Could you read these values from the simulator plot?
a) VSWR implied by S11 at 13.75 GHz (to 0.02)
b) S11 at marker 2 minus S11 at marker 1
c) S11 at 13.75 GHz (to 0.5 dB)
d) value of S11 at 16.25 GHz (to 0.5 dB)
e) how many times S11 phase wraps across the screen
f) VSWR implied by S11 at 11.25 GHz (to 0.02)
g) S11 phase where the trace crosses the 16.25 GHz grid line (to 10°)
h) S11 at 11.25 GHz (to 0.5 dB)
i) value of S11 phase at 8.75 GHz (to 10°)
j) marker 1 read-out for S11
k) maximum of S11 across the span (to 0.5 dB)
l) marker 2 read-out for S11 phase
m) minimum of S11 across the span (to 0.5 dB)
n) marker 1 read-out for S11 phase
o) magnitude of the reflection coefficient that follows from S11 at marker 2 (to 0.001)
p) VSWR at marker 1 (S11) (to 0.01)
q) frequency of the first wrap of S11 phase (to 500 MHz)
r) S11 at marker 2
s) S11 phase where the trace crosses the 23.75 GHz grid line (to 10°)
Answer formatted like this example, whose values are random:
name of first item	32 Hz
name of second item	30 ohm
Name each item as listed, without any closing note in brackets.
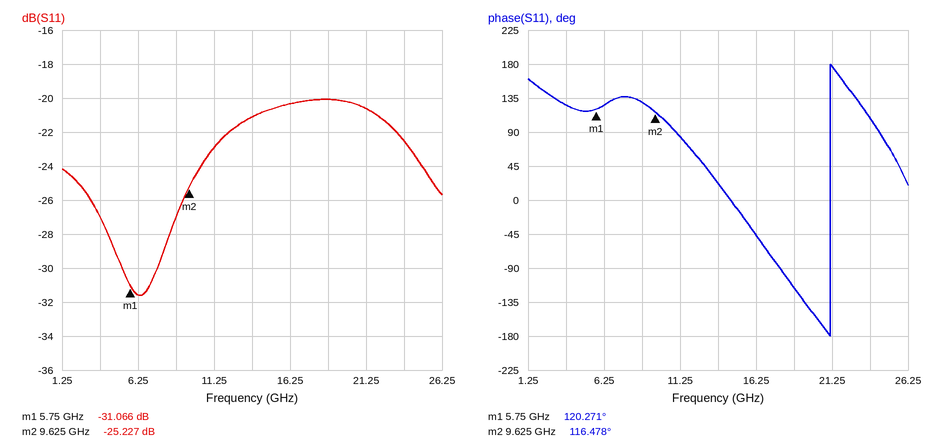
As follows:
VSWR implied by S11 at 13.75 GHz	1.20
S11 at marker 2 minus S11 at marker 1	5.839 dB
S11 at 13.75 GHz	-21.0 dB
value of S11 at 16.25 GHz	-20.5 dB
how many times S11 phase wraps across the screen	1
VSWR implied by S11 at 11.25 GHz	1.16
S11 phase where the trace crosses the 16.25 GHz grid line	-50°
S11 at 11.25 GHz	-23.0 dB
value of S11 phase at 8.75 GHz	130°
marker 1 read-out for S11	-31.066 dB
maximum of S11 across the span	-20.0 dB
marker 2 read-out for S11 phase	116.478°
minimum of S11 across the span	-31.5 dB
marker 1 read-out for S11 phase	120.271°
magnitude of the reflection coefficient that follows from S11 at marker 2	0.055
VSWR at marker 1 (S11)	1.06
frequency of the first wrap of S11 phase	21.0 GHz
S11 at marker 2	-25.227 dB
S11 phase where the trace crosses the 23.75 GHz grid line	110°
